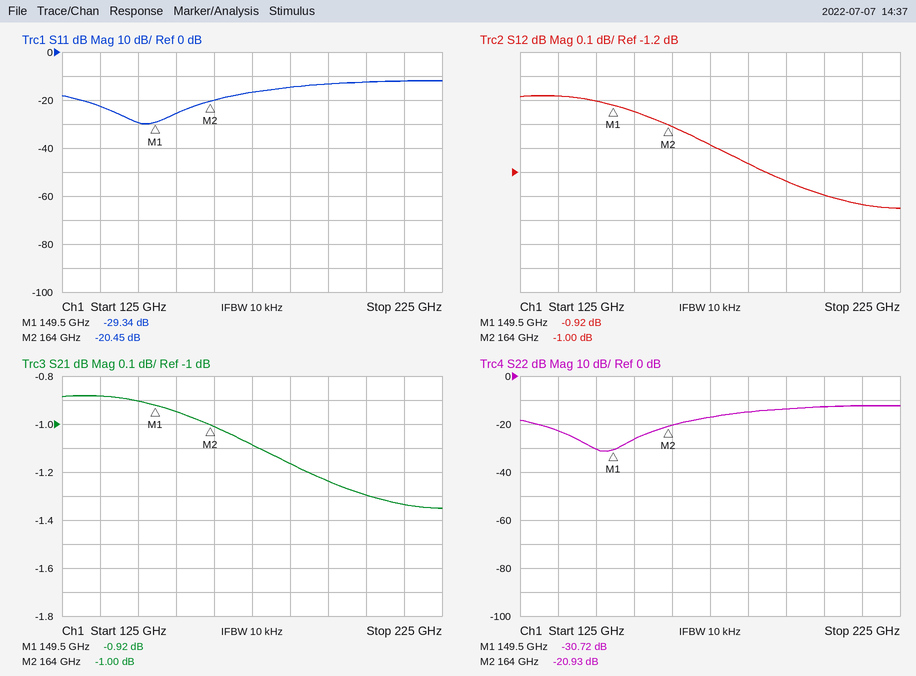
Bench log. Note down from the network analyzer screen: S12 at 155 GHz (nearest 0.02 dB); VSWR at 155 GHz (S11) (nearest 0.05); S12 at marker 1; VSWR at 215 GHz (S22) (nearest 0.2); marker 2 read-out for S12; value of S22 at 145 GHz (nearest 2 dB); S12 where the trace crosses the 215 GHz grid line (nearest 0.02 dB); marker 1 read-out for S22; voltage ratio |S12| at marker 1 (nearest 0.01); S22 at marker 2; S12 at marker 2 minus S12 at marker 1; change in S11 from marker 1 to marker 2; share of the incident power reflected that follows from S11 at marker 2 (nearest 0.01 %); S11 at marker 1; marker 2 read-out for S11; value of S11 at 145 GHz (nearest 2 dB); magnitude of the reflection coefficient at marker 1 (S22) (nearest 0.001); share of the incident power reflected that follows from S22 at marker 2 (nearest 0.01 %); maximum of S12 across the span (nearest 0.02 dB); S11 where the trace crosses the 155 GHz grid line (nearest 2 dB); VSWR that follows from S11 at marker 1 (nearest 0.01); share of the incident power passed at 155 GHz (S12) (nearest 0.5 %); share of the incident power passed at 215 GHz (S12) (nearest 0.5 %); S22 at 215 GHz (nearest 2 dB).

-0.94 dB
1.10
-0.92 dB
1.6
-1.00 dB
-30 dB
-1.34 dB
-30.72 dB
0.90
-20.93 dB
-0.08 dB
8.89 dB
0.90 %
-29.34 dB
-20.45 dB
-30 dB
0.029
0.81 %
-0.88 dB
-26 dB
1.07
80.5 %
73.5 %
-12 dB
